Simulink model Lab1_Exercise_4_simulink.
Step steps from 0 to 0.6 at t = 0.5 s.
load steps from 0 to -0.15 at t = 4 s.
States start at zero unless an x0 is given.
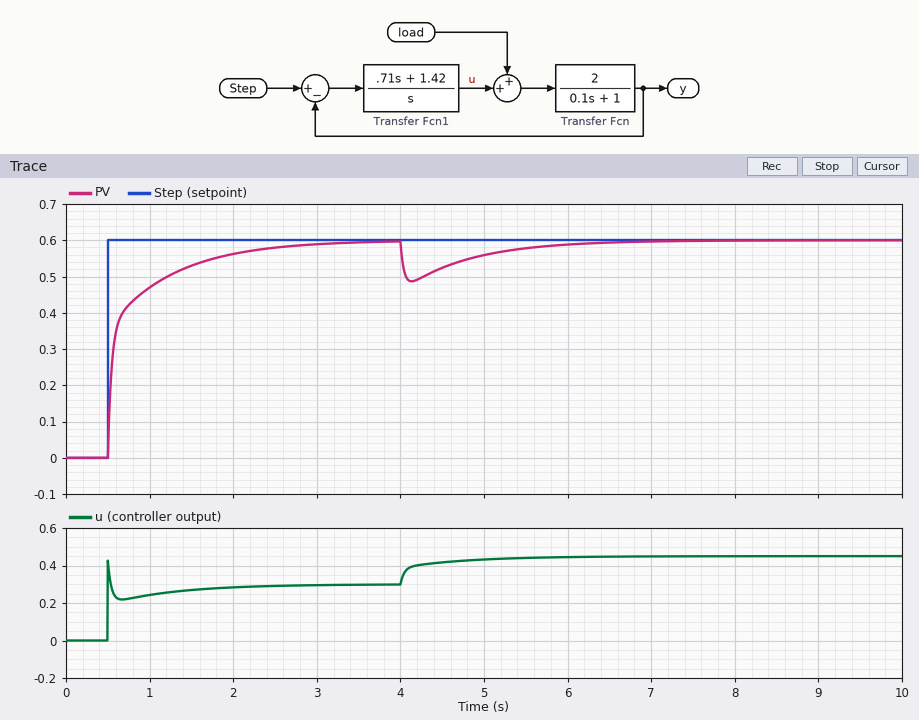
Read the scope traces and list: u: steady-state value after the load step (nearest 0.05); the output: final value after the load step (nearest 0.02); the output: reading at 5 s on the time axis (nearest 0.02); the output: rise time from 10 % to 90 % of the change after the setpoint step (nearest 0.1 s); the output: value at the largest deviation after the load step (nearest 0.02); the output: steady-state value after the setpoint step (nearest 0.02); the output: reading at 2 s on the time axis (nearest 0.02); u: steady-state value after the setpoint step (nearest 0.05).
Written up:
0.45
0.60
0.56
1.1 s
0.48
0.60
0.56
0.30
